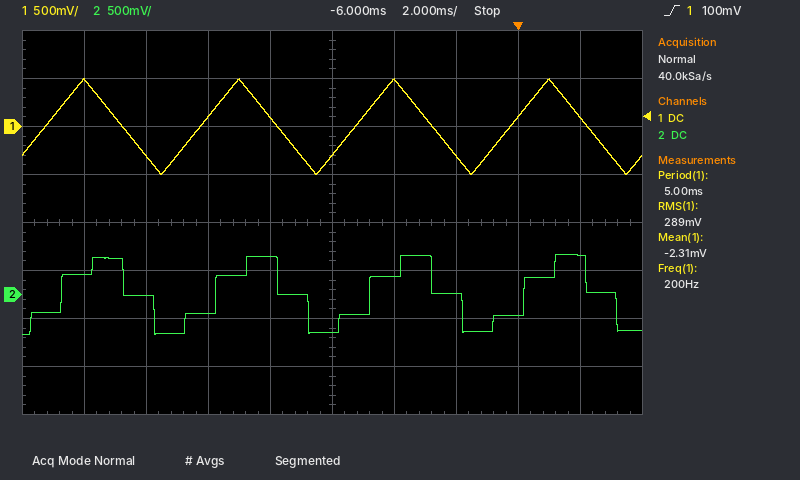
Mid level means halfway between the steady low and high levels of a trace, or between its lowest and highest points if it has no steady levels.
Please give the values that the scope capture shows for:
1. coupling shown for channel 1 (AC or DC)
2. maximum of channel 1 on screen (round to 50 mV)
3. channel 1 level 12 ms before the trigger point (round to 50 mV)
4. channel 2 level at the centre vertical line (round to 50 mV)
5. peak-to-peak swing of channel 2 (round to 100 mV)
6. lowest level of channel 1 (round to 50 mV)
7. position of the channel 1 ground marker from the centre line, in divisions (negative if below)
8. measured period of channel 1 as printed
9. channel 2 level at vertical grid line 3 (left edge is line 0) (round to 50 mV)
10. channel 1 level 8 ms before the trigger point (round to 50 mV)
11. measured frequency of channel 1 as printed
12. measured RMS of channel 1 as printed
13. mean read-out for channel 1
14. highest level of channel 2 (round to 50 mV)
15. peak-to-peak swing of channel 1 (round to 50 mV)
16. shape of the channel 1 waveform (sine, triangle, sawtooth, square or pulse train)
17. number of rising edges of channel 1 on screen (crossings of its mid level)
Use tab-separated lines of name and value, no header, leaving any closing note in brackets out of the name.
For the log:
coupling shown for channel 1	DC
maximum of channel 1 on screen	500 mV
channel 1 level 12 ms before the trigger point	-300 mV
channel 2 level at the centre vertical line	-400 mV
peak-to-peak swing of channel 2	800 mV
lowest level of channel 1	-500 mV
position of the channel 1 ground marker from the centre line, in divisions	+2.0 div
measured period of channel 1 as printed	5.00 ms
channel 2 level at vertical grid line 3 (left edge is line 0)	-200 mV
channel 1 level 8 ms before the trigger point	100 mV
measured frequency of channel 1 as printed	200 Hz
measured RMS of channel 1 as printed	289 mV
mean read-out for channel 1	-2.31 mV
highest level of channel 2	400 mV
peak-to-peak swing of channel 1	1.00 V
shape of the channel 1 waveform	triangle
number of rising edges of channel 1 on screen	4
